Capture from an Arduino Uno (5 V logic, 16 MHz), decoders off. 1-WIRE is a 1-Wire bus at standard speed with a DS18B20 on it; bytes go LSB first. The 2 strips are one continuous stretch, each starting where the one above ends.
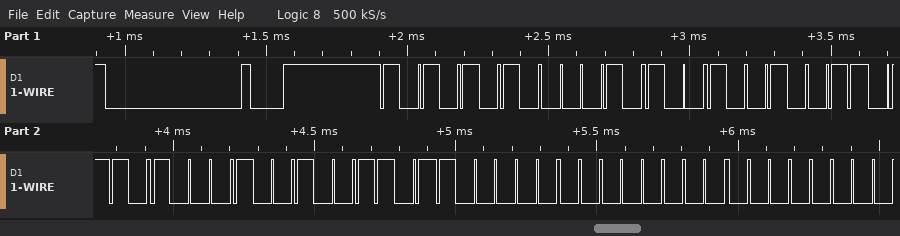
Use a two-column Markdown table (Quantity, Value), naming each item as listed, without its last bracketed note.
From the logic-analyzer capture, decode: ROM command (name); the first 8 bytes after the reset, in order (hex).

| Quantity | Value |
|---|---|
| ROM command | Match ROM |
| the first 8 bytes after the reset, in order | 55 28 C9 16 C9 06 00 00 |
